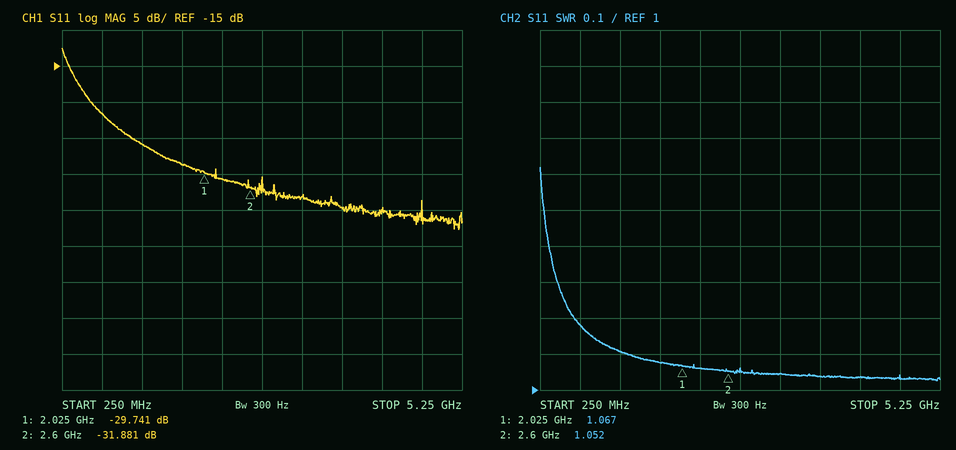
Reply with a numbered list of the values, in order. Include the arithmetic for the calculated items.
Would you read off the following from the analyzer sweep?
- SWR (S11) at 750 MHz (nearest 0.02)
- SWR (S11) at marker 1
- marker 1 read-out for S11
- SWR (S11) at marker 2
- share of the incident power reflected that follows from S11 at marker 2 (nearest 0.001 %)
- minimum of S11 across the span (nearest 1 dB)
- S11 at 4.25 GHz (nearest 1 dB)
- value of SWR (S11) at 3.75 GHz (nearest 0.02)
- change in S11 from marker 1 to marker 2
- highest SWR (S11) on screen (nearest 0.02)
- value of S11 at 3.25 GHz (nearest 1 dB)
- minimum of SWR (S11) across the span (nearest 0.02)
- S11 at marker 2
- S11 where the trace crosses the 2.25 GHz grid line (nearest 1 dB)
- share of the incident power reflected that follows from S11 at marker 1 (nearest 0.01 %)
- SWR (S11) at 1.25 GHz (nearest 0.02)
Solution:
1. 1.18
2. 1.067
3. -29.741 dB
4. 1.052
5. 10^(-31.881/10) ≈ 0.065 %
6. -38 dB
7. -35 dB
8. 1.04
9. -31.881 − (-29.741) = -2.140 dB
10. 1.62
11. -33 dB
12. 1.02
13. -31.881 dB
14. -31 dB
15. 10^(-29.741/10) ≈ 0.11 %
16. 1.10
